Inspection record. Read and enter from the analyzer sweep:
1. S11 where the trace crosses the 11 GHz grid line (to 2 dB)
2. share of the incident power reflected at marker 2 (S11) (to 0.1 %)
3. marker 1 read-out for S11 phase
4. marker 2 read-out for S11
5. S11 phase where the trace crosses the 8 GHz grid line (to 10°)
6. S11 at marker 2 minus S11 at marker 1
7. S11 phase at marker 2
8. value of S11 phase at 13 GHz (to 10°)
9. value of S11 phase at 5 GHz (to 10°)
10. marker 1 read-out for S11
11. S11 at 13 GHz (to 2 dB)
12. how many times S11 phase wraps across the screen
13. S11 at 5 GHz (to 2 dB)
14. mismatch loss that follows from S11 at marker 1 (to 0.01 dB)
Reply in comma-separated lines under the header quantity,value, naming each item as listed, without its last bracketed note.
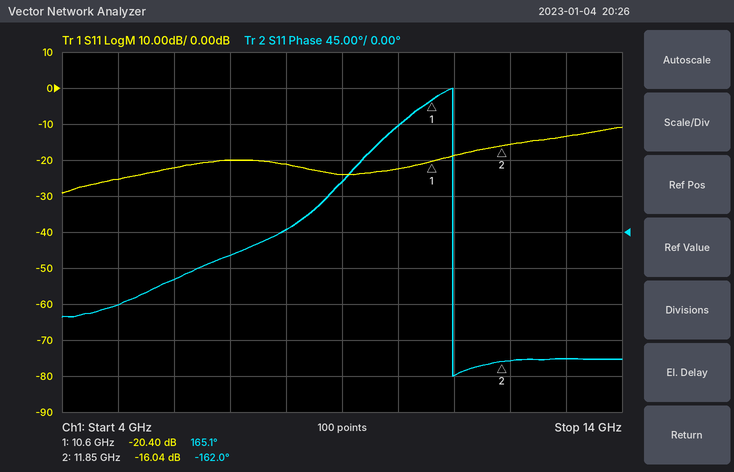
quantity,value
S11 where the trace crosses the 11 GHz grid line,-18 dB
share of the incident power reflected at marker 2 (S11),2.5 %
marker 1 read-out for S11 phase,165.1°
marker 2 read-out for S11,-16.04 dB
S11 phase where the trace crosses the 8 GHz grid line,0°
S11 at marker 2 minus S11 at marker 1,4.36 dB
S11 phase at marker 2,-162.0°
value of S11 phase at 13 GHz,-160°
value of S11 phase at 5 GHz,-90°
marker 1 read-out for S11,-20.40 dB
S11 at 13 GHz,-14 dB
how many times S11 phase wraps across the screen,1
S11 at 5 GHz,-26 dB
mismatch loss that follows from S11 at marker 1,0.04 dB
